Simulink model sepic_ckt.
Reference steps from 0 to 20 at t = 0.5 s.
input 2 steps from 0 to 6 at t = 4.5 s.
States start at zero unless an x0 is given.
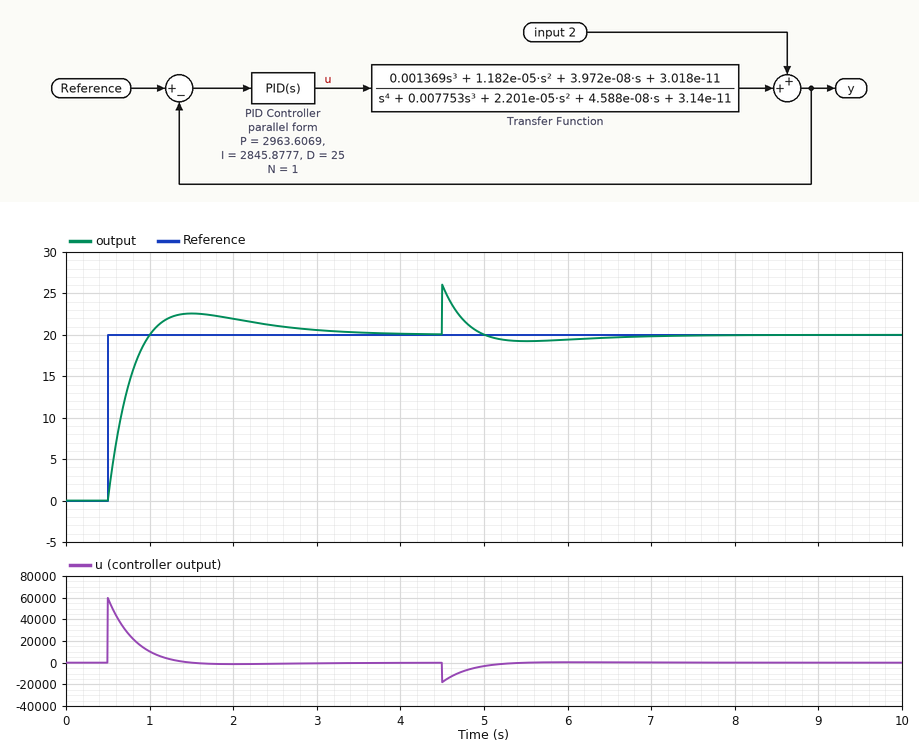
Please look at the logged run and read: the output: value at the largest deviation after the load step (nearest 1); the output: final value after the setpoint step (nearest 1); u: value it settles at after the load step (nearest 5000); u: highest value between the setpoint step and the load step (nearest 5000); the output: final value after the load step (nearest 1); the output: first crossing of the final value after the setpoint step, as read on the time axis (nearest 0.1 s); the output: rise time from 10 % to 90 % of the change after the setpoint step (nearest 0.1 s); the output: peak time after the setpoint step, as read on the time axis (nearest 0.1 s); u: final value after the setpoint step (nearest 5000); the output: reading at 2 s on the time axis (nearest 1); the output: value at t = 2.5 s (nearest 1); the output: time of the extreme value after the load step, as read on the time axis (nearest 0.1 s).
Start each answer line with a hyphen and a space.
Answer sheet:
- 26
- 20
- 0
- 60000
- 20
- 1.0 s
- 0.4 s
- 1.5 s
- 0
- 22
- 21
- 4.5 s
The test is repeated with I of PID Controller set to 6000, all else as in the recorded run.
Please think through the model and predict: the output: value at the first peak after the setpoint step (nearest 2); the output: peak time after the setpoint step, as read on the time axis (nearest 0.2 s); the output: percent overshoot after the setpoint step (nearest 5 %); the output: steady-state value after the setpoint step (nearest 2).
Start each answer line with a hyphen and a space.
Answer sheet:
- 24
- 1.2 s
- 20 %
- 20
